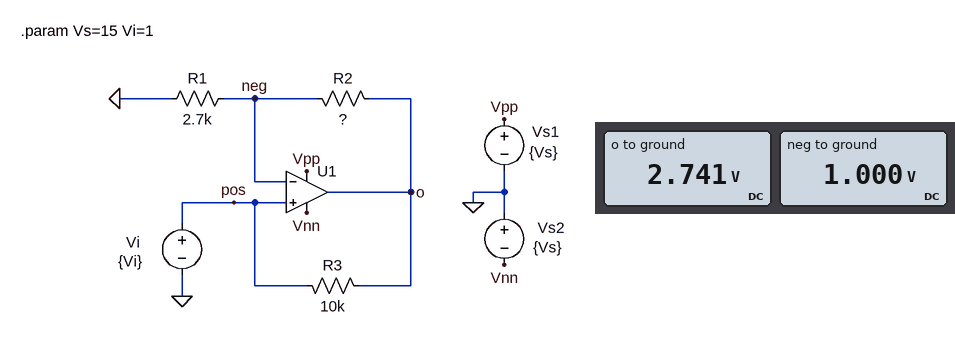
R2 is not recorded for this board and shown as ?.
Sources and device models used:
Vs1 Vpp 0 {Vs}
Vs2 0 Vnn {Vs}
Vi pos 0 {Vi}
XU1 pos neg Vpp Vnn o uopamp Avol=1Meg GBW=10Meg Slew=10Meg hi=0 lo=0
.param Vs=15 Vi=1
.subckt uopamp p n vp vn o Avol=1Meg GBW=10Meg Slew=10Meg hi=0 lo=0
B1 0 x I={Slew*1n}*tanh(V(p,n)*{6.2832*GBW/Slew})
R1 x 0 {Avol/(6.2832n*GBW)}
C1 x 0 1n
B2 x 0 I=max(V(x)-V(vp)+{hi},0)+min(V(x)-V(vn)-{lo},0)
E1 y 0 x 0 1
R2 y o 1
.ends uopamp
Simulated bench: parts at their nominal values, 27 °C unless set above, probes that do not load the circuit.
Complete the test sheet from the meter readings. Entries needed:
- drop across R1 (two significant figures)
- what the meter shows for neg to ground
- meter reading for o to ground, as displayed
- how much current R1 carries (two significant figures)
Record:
1.0 V
1.000 V
2.741 V
370 µA
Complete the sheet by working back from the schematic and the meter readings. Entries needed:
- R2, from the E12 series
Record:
4.7 kΩ
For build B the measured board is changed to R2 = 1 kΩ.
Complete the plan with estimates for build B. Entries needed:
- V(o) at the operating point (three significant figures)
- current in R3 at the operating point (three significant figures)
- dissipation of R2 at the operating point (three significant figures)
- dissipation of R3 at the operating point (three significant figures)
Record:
1.37 V
37.0 µA
137 µW
13.7 µW
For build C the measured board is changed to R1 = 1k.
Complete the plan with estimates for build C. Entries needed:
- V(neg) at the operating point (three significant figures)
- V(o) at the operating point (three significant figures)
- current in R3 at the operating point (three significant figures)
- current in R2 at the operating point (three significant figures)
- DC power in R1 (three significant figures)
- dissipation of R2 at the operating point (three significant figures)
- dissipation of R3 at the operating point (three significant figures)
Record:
1.00 V
5.70 V
470 µA
1.00 mA
1.00 mW
4.70 mW
2.21 mW
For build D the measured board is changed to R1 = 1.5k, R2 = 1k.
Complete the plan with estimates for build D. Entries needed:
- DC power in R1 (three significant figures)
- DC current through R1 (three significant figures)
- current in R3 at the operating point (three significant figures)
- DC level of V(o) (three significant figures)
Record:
667 µW
667 µA
66.7 µA
1.67 V
